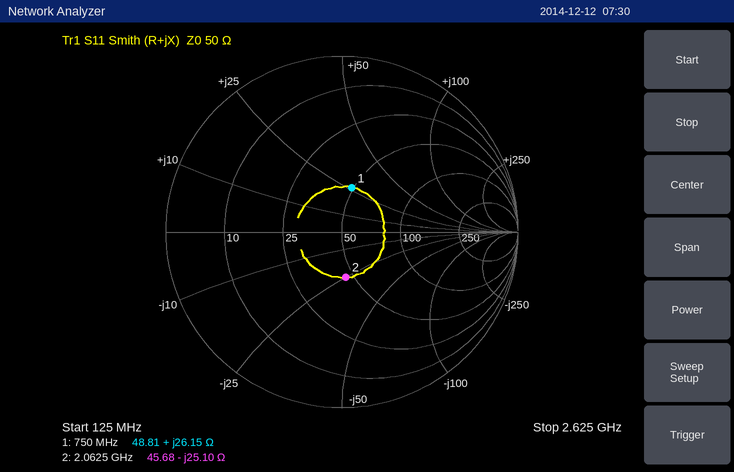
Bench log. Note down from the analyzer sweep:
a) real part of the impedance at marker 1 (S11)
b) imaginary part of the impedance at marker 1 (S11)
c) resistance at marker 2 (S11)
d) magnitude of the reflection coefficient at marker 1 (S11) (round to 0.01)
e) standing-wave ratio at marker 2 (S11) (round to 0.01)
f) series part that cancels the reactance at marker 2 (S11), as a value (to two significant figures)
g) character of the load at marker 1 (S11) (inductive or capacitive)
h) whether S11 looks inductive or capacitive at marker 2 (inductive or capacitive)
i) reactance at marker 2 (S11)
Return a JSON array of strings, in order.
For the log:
["48.81 Ω", "+26.15 Ω", "45.68 Ω", "0.26", "1.69", "1.9 nH", "inductive", "capacitive", "-25.10 Ω"]
